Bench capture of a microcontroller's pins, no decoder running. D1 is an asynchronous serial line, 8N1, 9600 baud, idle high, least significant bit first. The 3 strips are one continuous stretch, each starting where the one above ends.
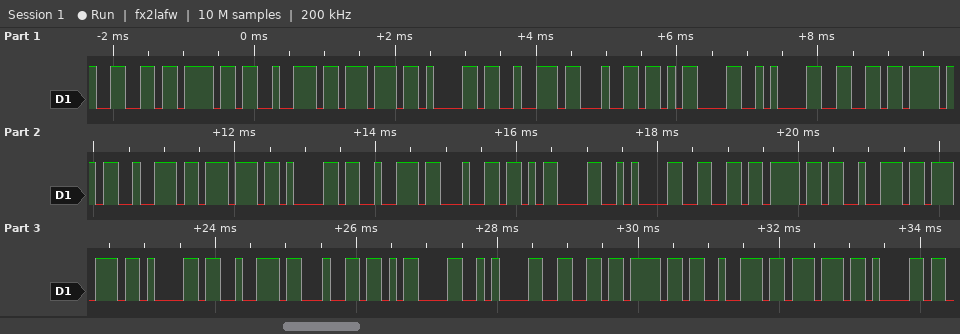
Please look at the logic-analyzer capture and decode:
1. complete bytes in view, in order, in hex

66 6F 72 77 61 72 64 0D 0A 66 6F 72 77 61 72 64 0D 0A 66 6F 72 77 61 72 64 0D 0A 66 6F 72 77 61
